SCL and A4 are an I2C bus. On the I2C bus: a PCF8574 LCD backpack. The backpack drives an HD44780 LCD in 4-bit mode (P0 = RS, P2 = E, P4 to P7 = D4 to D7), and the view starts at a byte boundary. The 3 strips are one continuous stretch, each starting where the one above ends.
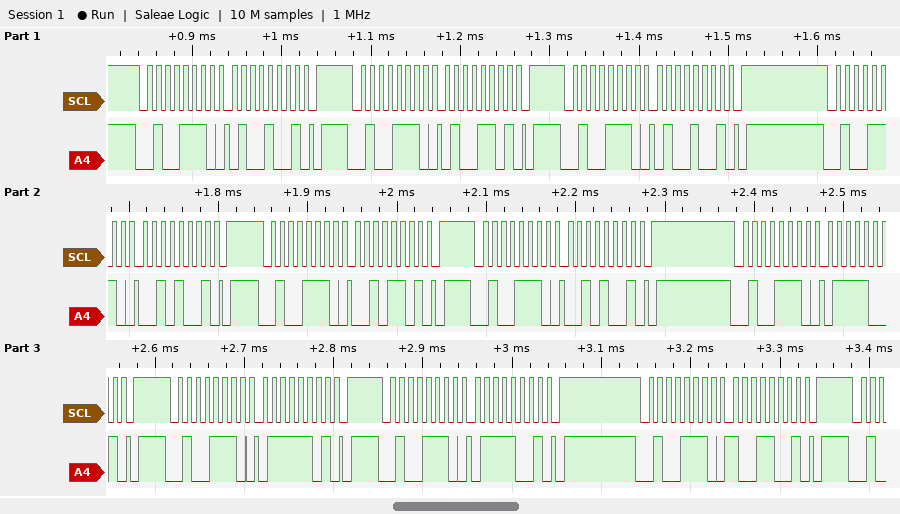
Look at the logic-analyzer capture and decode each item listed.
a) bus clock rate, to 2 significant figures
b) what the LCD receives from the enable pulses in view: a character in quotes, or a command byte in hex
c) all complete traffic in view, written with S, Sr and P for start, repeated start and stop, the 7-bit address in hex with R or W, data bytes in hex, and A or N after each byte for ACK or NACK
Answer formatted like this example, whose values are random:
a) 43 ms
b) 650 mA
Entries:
a) 100 kHz
b) 'B'
c) S 27W A 49 A P S 27W A 4D A P S 27W A 49 A P S 27W A 29 A P S 27W A 2D A P S 27W A 29 A P S 27W A 79 A P S 27W A 7D A P S 27W A 79 A P S 27W A 99 A P
